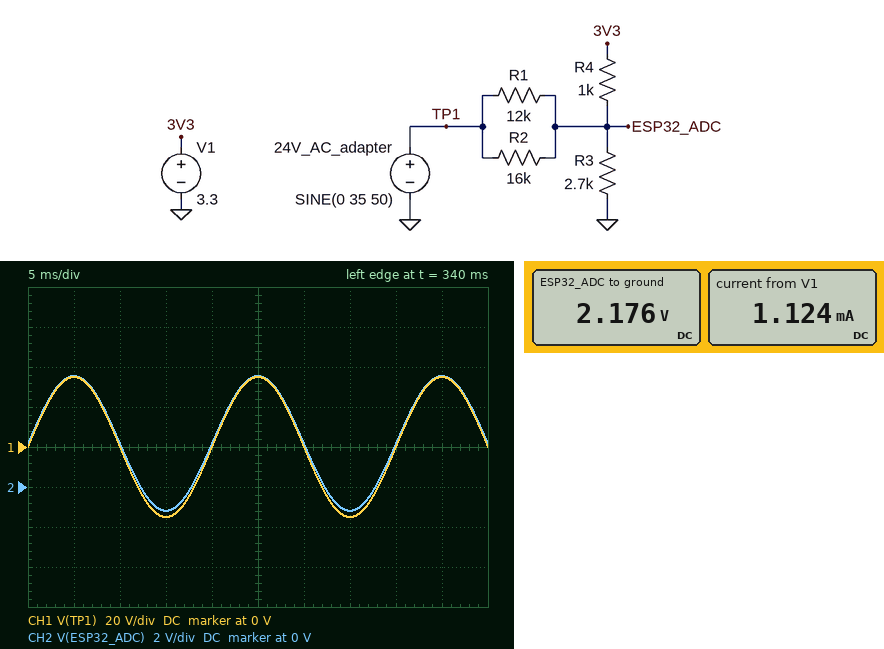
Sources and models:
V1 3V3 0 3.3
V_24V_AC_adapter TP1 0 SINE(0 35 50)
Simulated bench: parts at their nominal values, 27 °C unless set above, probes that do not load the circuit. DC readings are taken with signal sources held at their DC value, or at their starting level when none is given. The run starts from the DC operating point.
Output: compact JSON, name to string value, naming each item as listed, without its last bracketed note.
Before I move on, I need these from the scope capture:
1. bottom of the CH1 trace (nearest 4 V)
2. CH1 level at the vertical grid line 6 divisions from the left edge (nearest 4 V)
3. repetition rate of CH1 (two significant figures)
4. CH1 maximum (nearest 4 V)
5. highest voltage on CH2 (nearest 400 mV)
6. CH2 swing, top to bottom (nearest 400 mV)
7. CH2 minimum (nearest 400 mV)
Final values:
{"bottom of the CH1 trace": "-36 V", "CH1 level at the vertical grid line 6 divisions from the left edge": "0 V", "repetition rate of CH1": "50 Hz", "CH1 maximum": "36 V", "highest voltage on CH2": "5.6 V", "CH2 swing, top to bottom": "6.8 V", "CH2 minimum": "-1.2 V"}
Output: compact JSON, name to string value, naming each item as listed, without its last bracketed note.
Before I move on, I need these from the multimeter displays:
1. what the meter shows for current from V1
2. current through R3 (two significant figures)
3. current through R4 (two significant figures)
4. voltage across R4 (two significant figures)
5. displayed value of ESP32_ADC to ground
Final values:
{"what the meter shows for current from V1": "1.124 mA", "current through R3": "810 µA", "current through R4": "1.1 mA", "voltage across R4": "1.1 V", "displayed value of ESP32_ADC to ground": "2.176 V"}
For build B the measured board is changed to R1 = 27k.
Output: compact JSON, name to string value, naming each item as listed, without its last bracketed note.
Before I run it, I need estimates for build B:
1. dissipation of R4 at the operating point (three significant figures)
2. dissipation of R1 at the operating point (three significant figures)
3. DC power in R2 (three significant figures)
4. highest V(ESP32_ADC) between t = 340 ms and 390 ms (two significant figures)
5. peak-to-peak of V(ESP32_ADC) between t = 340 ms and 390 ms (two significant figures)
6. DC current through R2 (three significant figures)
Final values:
{"dissipation of R4 at the operating point": "1.11 mW", "dissipation of R1 at the operating point": "187 µW", "DC power in R2": "315 µW", "highest V(ESP32_ADC) between t = 340 ms and 390 ms": "4.6 V", "peak-to-peak of V(ESP32_ADC) between t = 340 ms and 390 ms": "4.7 V", "DC current through R2": "140 µA"}
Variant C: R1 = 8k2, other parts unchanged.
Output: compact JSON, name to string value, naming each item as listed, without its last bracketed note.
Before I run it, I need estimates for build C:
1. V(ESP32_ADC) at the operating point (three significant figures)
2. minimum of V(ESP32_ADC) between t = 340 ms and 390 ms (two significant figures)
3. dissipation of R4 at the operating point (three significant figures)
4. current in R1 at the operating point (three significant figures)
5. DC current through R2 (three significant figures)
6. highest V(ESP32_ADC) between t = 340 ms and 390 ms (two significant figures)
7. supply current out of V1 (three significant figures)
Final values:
{"V(ESP32_ADC) at the operating point": "2.12 V", "minimum of V(ESP32_ADC) between t = 340 ms and 390 ms": "-2.0 V", "dissipation of R4 at the operating point": "1.39 mW", "current in R1 at the operating point": "259 µA", "DC current through R2": "133 µA", "highest V(ESP32_ADC) between t = 340 ms and 390 ms": "6.3 V", "supply current out of V1": "1.18 mA"}
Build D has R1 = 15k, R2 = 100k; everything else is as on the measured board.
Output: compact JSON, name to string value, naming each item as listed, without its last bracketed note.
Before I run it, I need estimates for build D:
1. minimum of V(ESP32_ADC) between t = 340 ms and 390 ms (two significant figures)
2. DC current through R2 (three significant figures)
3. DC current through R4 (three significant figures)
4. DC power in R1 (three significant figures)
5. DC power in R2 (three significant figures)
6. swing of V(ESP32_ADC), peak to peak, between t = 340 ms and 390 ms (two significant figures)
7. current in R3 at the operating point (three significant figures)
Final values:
{"minimum of V(ESP32_ADC) between t = 340 ms and 390 ms": "430 mV", "DC current through R2": "22.8 µA", "DC current through R4": "1.02 mA", "DC power in R1": "347 µW", "DC power in R2": "52.0 µW", "swing of V(ESP32_ADC), peak to peak, between t = 340 ms and 390 ms": "3.7 V", "current in R3 at the operating point": "845 µA"}
